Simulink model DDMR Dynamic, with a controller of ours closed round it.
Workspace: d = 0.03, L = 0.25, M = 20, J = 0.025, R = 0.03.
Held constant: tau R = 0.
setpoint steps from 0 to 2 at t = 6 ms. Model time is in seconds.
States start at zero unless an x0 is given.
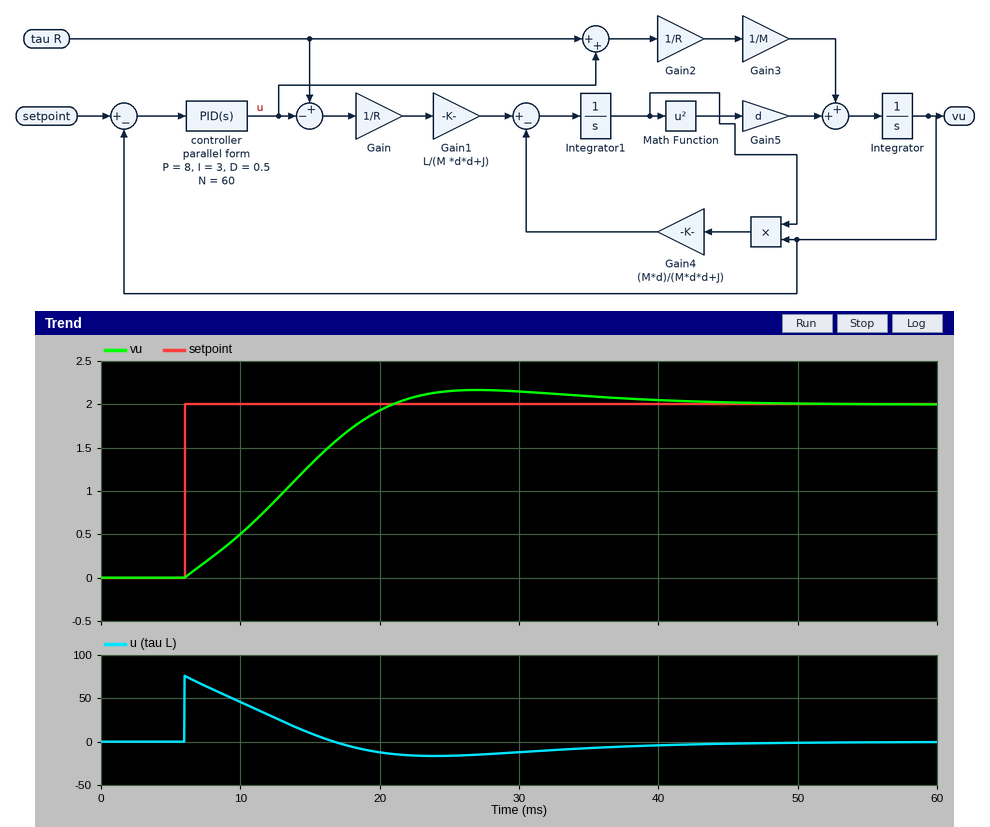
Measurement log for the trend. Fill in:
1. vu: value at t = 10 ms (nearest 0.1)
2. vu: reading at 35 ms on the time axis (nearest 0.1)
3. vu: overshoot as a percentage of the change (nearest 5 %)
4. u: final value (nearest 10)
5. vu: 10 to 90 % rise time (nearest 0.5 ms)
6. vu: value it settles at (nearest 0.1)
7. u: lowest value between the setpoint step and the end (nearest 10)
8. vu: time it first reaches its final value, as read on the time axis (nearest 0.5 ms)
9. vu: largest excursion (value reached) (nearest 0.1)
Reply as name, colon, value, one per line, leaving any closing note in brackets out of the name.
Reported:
vu: value at t = 10 ms: 0.5
vu: reading at 35 ms on the time axis: 2.1
vu: overshoot as a percentage of the change: 10 %
u: final value: 0
vu: 10 to 90 % rise time: 11.0 ms
vu: value it settles at: 2.0
u: lowest value between the setpoint step and the end: -20
vu: time it first reaches its final value, as read on the time axis: 21.0 ms
vu: largest excursion (value reached): 2.2
